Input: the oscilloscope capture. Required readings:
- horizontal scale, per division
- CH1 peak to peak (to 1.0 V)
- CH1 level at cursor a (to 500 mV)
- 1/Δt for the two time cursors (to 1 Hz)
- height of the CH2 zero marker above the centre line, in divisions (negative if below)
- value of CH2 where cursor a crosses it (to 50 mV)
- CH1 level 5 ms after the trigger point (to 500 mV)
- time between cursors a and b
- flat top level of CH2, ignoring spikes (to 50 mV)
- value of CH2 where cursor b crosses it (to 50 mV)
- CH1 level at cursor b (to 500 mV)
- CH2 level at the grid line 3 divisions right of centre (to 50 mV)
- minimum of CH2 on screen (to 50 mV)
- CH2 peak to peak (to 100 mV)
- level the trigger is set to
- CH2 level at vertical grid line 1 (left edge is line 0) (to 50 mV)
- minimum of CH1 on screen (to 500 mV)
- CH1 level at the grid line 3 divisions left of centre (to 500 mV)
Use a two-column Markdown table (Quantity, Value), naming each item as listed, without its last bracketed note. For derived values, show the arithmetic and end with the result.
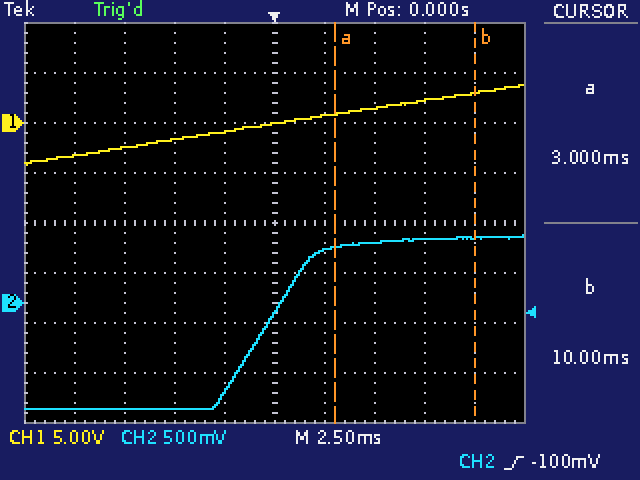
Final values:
| Quantity | Value |
|---|---|
| horizontal scale, per division | 2.5 ms |
| CH1 peak to peak | 8.0 V |
| CH1 level at cursor a | 1.0 V |
| 1/Δt for the two time cursors | 1 / 7.00 ms ≈ 143 Hz |
| height of the CH2 zero marker above the centre line, in divisions | -1.6 div |
| value of CH2 where cursor a crosses it | 550 mV |
| CH1 level 5 ms after the trigger point | 1.5 V |
| time between cursors a and b | 10 ms − (3 ms) = 7.00 ms |
| flat top level of CH2, ignoring spikes | 650 mV |
| value of CH2 where cursor b crosses it | 650 mV |
| CH1 level at cursor b | 3.0 V |
| CH2 level at the grid line 3 divisions right of centre | 650 mV |
| minimum of CH2 on screen | -1.05 V |
| CH2 peak to peak | 1.70 V |
| level the trigger is set to | -100 mV |
| CH2 level at vertical grid line 1 (left edge is line 0) | -1.05 V |
| minimum of CH1 on screen | -4.0 V |
| CH1 level at the grid line 3 divisions left of centre | -2.5 V |
